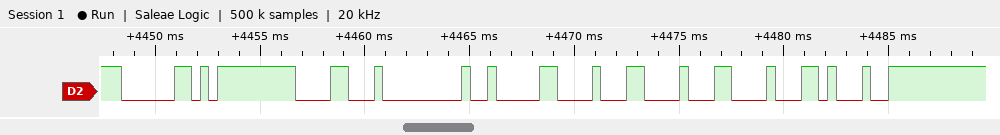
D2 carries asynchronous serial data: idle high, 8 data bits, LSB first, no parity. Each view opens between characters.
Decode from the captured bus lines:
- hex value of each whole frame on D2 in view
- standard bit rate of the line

60, FF, 18, 00, 82, 88, 88, 88, 91
2400 baud
